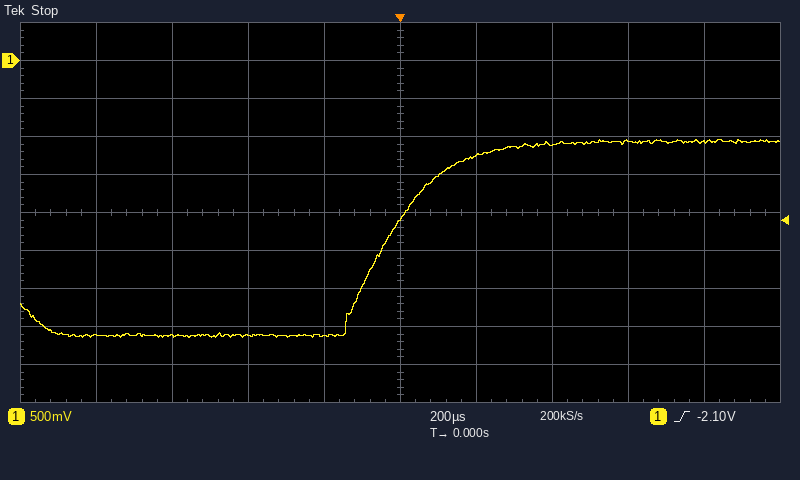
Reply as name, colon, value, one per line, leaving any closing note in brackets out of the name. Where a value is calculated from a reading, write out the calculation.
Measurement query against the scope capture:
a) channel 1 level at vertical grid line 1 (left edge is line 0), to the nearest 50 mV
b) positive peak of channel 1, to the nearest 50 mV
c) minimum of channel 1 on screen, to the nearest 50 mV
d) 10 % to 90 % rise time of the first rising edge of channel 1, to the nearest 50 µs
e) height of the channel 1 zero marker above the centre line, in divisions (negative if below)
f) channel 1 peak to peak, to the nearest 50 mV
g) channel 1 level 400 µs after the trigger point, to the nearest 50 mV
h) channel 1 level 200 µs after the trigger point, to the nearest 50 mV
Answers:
channel 1 level at vertical grid line 1 (left edge is line 0), to the nearest 50 mV: -3.60 V
positive peak of channel 1, to the nearest 50 mV: -1.05 V
minimum of channel 1 on screen, to the nearest 50 mV: -3.65 V
10 % to 90 % rise time of the first rising edge of channel 1, to the nearest 50 µs: 300 µs
height of the channel 1 zero marker above the centre line, in divisions: +4.0 div
channel 1 peak to peak, to the nearest 50 mV: -1.05 V − (-3.65 V) = 2.60 V
channel 1 level 400 µs after the trigger point, to the nearest 50 mV: -1.10 V
channel 1 level 200 µs after the trigger point, to the nearest 50 mV: -1.25 V
